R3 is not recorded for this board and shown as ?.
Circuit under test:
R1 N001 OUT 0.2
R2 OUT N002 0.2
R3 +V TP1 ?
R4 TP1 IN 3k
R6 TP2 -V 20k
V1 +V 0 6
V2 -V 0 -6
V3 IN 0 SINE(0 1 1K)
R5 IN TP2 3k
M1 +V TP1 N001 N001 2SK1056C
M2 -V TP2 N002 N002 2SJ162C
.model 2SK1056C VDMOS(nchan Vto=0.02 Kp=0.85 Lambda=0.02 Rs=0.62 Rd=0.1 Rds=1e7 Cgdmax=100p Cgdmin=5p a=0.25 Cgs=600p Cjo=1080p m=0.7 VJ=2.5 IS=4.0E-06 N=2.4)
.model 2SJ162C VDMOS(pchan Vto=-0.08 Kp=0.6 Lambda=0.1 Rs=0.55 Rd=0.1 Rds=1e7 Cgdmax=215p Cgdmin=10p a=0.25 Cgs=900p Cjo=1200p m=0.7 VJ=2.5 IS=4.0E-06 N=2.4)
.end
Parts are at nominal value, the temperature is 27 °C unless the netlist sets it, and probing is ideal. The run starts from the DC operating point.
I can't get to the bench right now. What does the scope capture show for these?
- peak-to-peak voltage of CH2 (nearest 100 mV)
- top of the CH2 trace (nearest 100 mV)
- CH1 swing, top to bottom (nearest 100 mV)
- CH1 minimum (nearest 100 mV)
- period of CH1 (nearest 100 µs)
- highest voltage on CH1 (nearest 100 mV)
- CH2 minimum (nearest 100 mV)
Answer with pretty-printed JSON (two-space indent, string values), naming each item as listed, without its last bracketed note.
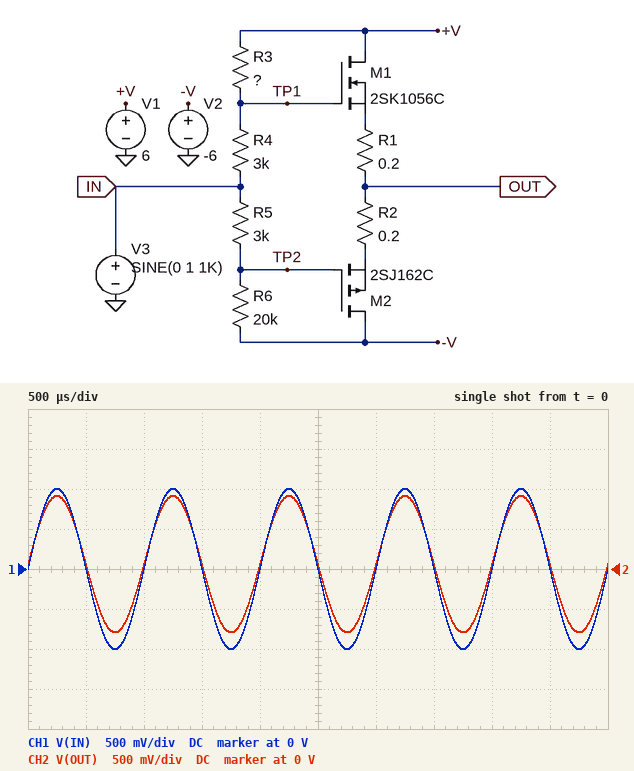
{
  "peak-to-peak voltage of CH2": "1.7 V",
  "top of the CH2 trace": "900 mV",
  "CH1 swing, top to bottom": "2.0 V",
  "CH1 minimum": "-1.0 V",
  "period of CH1": "1.0 ms",
  "highest voltage on CH1": "1.0 V",
  "CH2 minimum": "-800 mV"
}
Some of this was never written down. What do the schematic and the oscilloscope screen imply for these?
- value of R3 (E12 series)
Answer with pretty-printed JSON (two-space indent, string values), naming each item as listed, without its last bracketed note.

{
  "value of R3": "18 kΩ"
}
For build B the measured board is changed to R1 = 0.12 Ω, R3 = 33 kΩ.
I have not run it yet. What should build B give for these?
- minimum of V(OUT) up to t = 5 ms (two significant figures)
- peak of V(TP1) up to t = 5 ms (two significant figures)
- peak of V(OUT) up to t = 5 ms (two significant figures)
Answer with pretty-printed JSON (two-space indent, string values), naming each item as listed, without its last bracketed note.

{
  "minimum of V(OUT) up to t = 5 ms": "-990 mV",
  "peak of V(TP1) up to t = 5 ms": "1.4 V",
  "peak of V(OUT) up to t = 5 ms": "770 mV"
}
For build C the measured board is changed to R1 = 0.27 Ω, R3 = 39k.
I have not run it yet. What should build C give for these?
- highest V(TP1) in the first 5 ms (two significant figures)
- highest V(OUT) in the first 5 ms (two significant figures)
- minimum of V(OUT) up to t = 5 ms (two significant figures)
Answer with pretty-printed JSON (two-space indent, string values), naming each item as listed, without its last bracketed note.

{
  "highest V(TP1) in the first 5 ms": "1.4 V",
  "highest V(OUT) in the first 5 ms": "740 mV",
  "minimum of V(OUT) up to t = 5 ms": "-1.0 V"
}
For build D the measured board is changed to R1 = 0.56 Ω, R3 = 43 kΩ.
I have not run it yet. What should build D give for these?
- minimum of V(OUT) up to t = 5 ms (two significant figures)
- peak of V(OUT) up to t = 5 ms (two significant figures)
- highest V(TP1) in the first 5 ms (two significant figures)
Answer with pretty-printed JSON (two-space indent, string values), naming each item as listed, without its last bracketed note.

{
  "minimum of V(OUT) up to t = 5 ms": "-1.1 V",
  "peak of V(OUT) up to t = 5 ms": "710 mV",
  "highest V(TP1) in the first 5 ms": "1.3 V"
}
